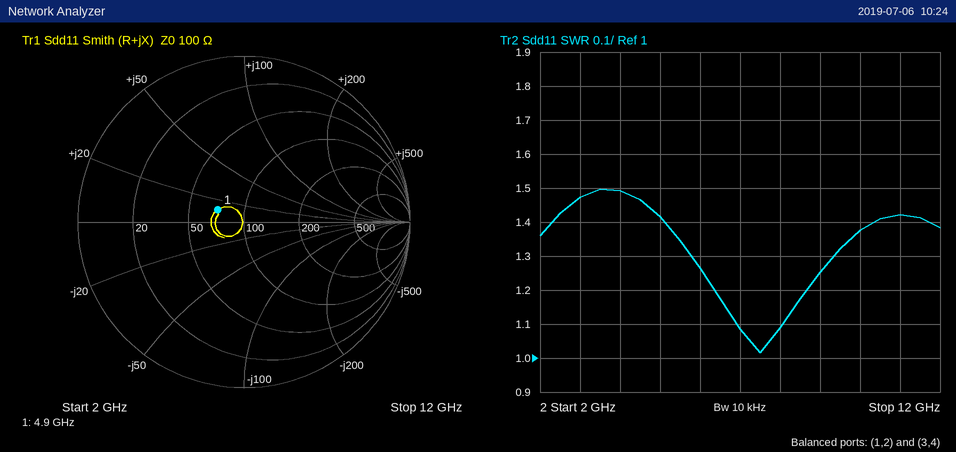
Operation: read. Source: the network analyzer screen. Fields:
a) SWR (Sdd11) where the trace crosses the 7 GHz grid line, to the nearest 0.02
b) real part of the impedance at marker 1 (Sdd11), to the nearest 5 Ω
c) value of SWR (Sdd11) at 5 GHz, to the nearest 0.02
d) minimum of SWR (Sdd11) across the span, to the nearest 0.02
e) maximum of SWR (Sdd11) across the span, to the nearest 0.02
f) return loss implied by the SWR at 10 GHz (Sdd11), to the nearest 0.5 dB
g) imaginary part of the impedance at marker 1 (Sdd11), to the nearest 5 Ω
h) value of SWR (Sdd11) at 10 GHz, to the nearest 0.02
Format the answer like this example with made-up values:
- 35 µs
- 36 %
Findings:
- 1.08
- 70 Ω
- 1.42
- 1.02
- 1.50
- 16.0 dB
- +10 Ω
- 1.38
